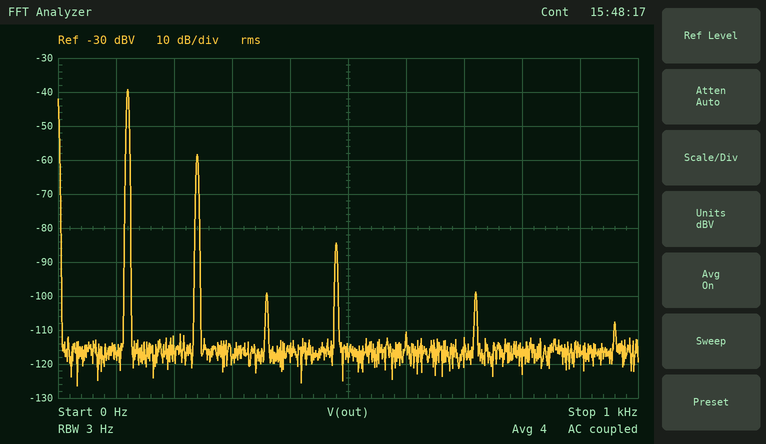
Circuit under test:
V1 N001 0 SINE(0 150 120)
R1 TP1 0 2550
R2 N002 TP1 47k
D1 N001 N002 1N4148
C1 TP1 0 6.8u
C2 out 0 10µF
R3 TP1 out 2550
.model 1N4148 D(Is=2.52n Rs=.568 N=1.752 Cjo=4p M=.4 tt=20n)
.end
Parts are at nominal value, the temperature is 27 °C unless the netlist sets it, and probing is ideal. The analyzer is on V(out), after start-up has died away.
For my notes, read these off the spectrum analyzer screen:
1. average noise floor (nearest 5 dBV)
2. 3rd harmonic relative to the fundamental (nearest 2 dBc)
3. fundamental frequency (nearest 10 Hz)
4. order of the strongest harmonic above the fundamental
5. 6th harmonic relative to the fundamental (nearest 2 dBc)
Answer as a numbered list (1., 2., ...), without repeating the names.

1. -115 dBV
2. -60 dBc
3. 120 Hz
4. 2
5. -60 dBc
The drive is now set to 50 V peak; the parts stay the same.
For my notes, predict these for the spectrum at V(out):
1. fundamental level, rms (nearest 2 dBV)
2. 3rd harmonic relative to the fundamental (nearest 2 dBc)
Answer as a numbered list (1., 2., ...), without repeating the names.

1. -48 dBV
2. -58 dBc
